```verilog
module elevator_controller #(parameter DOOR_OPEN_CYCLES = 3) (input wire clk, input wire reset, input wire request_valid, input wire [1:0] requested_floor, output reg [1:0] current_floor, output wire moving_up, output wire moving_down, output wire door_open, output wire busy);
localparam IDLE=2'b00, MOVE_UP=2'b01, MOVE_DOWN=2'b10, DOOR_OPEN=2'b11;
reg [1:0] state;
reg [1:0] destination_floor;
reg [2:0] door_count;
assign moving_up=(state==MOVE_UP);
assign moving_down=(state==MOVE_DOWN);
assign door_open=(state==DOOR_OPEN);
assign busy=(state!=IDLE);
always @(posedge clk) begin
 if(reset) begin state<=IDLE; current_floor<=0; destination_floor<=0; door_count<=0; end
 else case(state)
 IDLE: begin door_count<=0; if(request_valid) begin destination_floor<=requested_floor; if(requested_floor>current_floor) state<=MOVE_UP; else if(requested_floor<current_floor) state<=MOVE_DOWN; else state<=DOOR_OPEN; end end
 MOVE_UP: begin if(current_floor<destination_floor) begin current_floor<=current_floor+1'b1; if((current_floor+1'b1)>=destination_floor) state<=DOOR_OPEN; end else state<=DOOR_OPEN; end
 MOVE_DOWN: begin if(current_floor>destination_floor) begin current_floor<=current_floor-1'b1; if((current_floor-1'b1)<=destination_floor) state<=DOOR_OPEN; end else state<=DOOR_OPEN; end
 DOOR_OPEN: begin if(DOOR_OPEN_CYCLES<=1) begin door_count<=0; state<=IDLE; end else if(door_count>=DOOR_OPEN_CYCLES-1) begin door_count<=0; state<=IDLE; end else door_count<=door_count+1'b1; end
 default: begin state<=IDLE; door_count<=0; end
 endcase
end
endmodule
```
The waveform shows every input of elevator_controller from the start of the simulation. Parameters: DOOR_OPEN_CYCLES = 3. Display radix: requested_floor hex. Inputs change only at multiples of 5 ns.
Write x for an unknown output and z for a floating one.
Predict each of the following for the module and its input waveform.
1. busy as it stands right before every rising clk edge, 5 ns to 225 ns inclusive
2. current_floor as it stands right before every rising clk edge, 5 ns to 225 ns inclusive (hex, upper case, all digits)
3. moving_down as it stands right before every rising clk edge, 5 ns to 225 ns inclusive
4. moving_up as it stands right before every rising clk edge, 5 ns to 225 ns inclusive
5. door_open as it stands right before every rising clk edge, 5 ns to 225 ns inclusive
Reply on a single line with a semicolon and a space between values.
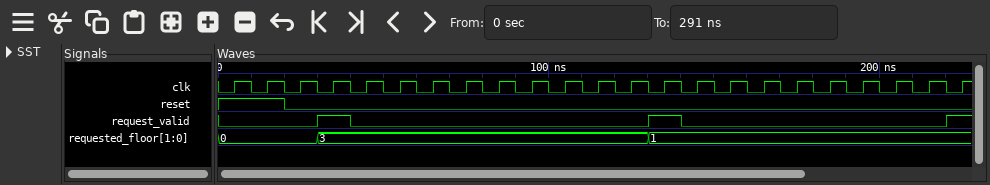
x 0 0 0 1 1 1 1 1 1 0 0 0 0 1 1 1 1 1 0 0 0 0; x, 0, 0, 0, 0, 1, 2, 3, 3, 3, 3, 3, 3, 3, 3, 2, 1, 1, 1, 1, 1, 1, 1; x 0 0 0 0 0 0 0 0 0 0 0 0 0 1 1 0 0 0 0 0 0 0; x 0 0 0 1 1 1 0 0 0 0 0 0 0 0 0 0 0 0 0 0 0 0; x 0 0 0 0 0 0 1 1 1 0 0 0 0 0 0 1 1 1 0 0 0 0
